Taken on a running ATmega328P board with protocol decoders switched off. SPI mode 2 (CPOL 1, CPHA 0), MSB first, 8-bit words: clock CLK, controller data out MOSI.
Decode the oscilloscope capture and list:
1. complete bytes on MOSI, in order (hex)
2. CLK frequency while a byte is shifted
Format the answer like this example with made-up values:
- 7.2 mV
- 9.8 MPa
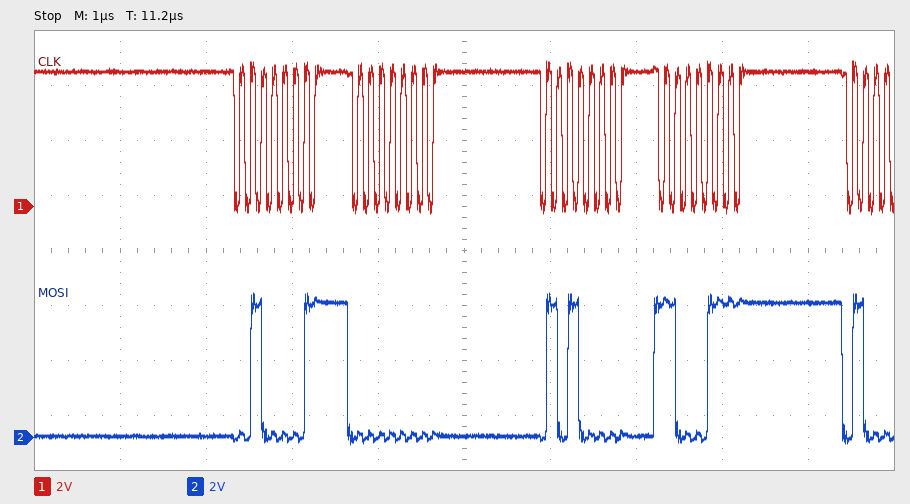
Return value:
- 0x21 0x00 0x50 0xC7
- 8 MHz
